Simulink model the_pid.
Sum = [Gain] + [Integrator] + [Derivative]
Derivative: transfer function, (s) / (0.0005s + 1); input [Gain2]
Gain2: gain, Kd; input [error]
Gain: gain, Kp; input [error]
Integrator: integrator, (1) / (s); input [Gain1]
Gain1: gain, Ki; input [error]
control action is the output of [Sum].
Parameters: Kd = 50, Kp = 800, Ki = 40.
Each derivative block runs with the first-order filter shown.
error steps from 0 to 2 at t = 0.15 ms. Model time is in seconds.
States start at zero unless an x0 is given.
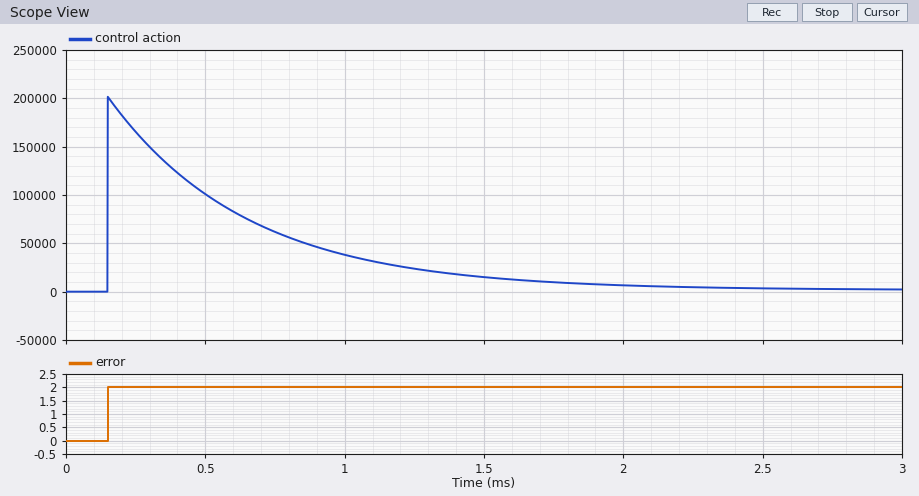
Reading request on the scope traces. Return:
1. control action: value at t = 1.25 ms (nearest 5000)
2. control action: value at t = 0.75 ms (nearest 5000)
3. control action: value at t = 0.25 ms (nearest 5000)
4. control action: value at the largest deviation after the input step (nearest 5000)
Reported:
25000
60000
165000
200000
